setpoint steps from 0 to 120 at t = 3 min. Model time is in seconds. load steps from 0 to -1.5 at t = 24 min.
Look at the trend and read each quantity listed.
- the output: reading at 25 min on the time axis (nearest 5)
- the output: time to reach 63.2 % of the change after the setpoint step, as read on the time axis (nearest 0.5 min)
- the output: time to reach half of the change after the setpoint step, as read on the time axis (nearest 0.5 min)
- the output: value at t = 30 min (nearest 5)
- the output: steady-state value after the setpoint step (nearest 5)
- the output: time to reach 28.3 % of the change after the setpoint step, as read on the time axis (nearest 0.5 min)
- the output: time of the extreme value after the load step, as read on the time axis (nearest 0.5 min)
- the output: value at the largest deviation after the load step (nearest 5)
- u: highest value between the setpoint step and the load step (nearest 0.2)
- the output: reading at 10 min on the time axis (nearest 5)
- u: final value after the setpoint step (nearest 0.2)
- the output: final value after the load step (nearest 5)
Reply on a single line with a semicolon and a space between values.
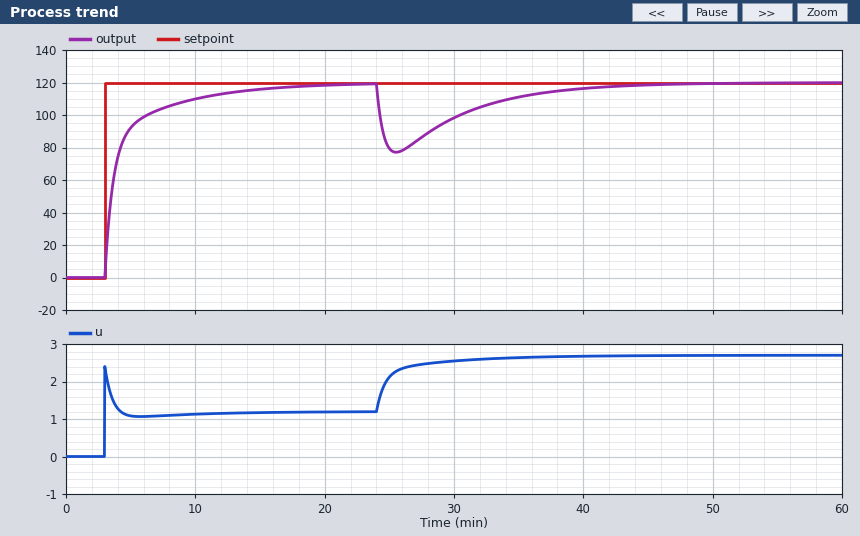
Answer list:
80; 4.0 min; 3.5 min; 100; 120; 3.5 min; 25.5 min; 75; 2.4; 110; 1.2; 120
